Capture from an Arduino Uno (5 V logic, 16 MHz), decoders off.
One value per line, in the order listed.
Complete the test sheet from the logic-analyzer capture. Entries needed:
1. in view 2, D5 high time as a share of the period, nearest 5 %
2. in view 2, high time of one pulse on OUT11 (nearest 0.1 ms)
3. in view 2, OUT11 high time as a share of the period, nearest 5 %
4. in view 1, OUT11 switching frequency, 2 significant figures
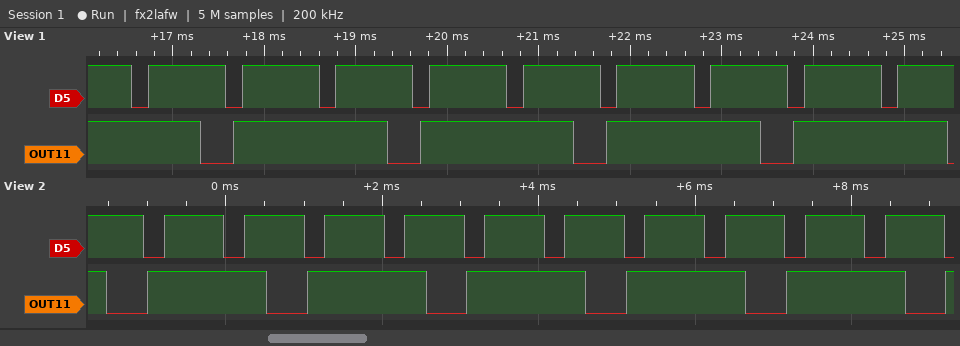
75 %
1.5 ms
75 %
490 Hz
